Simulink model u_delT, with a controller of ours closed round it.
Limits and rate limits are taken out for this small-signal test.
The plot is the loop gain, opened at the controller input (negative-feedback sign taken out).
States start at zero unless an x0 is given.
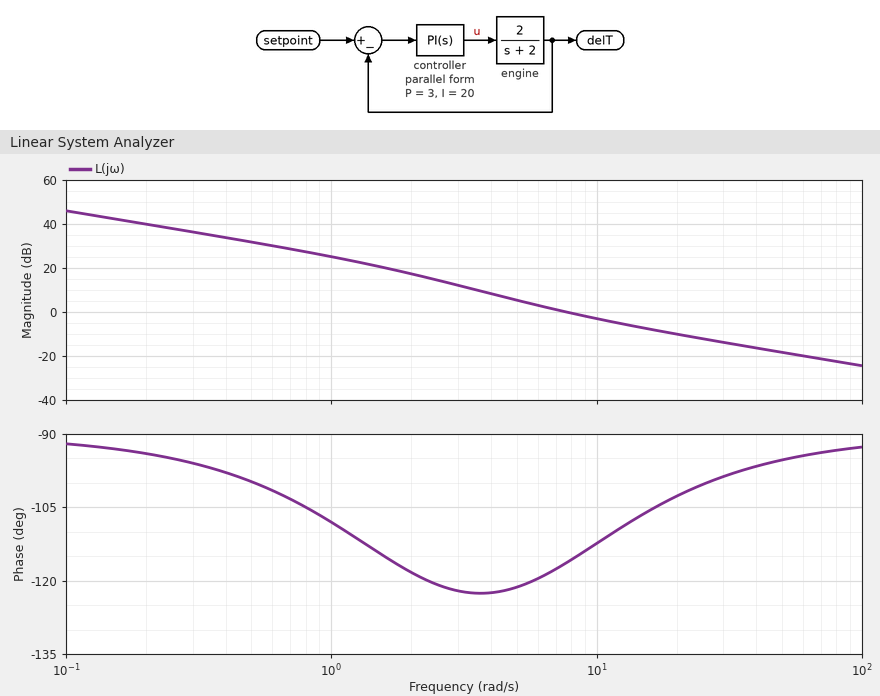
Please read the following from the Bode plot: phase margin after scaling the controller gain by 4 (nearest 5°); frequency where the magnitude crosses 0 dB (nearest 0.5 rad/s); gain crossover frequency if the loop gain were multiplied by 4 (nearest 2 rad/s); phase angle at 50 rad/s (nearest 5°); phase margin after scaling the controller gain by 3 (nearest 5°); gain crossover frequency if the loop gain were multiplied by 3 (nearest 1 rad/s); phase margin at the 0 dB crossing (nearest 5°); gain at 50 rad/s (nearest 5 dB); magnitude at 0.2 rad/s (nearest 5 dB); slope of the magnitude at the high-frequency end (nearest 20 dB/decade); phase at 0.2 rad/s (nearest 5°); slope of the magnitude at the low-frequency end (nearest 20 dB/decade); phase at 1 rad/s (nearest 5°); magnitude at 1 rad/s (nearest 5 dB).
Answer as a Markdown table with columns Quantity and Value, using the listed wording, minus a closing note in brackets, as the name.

| Quantity | Value |
|---|---|
| phase margin after scaling the controller gain by 4 | 80° |
| frequency where the magnitude crosses 0 dB | 7.5 rad/s |
| gain crossover frequency if the loop gain were multiplied by 4 | 24 rad/s |
| phase angle at 50 rad/s | -95° |
| phase margin after scaling the controller gain by 3 | 75° |
| gain crossover frequency if the loop gain were multiplied by 3 | 19 rad/s |
| phase margin at the 0 dB crossing | 65° |
| gain at 50 rad/s | -20 dB |
| magnitude at 0.2 rad/s | 40 dB |
| slope of the magnitude at the high-frequency end | -20 dB/decade |
| phase at 0.2 rad/s | -95° |
| slope of the magnitude at the low-frequency end | -20 dB/decade |
| phase at 1 rad/s | -110° |
| magnitude at 1 rad/s | 25 dB |
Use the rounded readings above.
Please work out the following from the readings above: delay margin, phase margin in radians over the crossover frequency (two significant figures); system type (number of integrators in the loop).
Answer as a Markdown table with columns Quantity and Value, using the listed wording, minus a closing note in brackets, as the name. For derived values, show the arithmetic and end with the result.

| Quantity | Value |
|---|---|
| delay margin, phase margin in radians over the crossover frequency | 65 × π / 180 / 7.5 = 0.15 s |
| system type | 1 |
